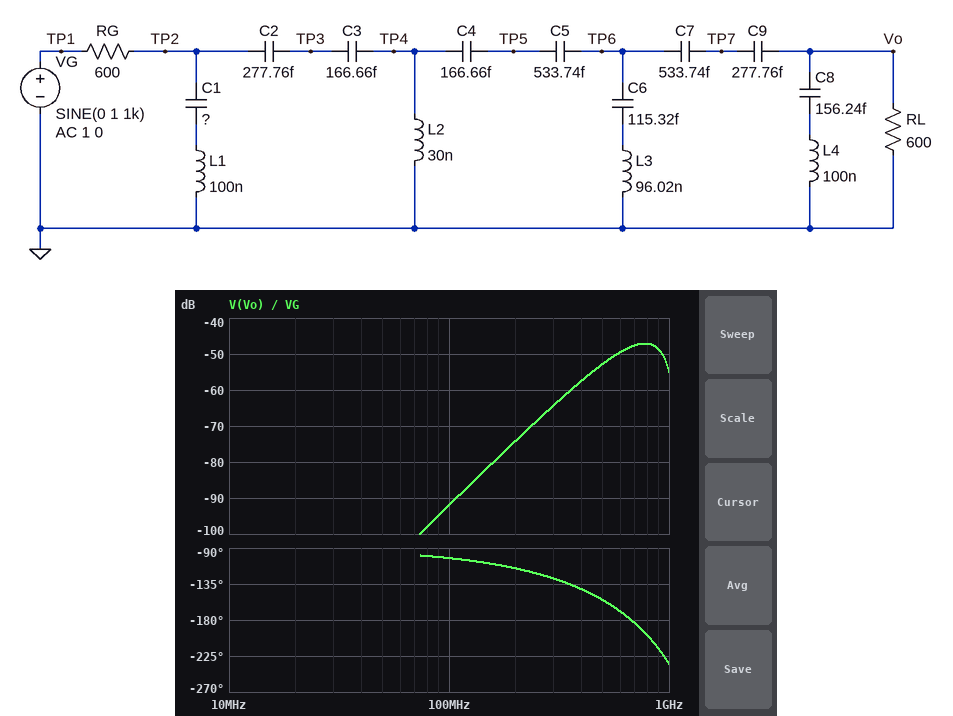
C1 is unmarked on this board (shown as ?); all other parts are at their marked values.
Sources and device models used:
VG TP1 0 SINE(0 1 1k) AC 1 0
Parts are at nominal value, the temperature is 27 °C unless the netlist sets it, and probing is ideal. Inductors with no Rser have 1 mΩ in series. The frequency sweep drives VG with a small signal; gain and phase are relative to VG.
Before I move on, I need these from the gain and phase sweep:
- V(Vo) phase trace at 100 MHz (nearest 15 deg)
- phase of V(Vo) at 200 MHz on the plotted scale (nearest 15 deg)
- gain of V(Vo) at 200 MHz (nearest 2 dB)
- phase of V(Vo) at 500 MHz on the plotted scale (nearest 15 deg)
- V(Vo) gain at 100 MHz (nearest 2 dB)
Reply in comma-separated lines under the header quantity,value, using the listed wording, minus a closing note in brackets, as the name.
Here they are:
quantity,value
V(Vo) phase trace at 100 MHz,-105 deg
phase of V(Vo) at 200 MHz on the plotted scale,-120 deg
gain of V(Vo) at 200 MHz,-74 dB
phase of V(Vo) at 500 MHz on the plotted scale,-150 deg
V(Vo) gain at 100 MHz,-92 dB
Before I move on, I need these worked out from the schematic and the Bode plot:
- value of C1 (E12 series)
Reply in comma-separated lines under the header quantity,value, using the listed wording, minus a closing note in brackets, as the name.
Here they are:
quantity,value
value of C1,220 fF
